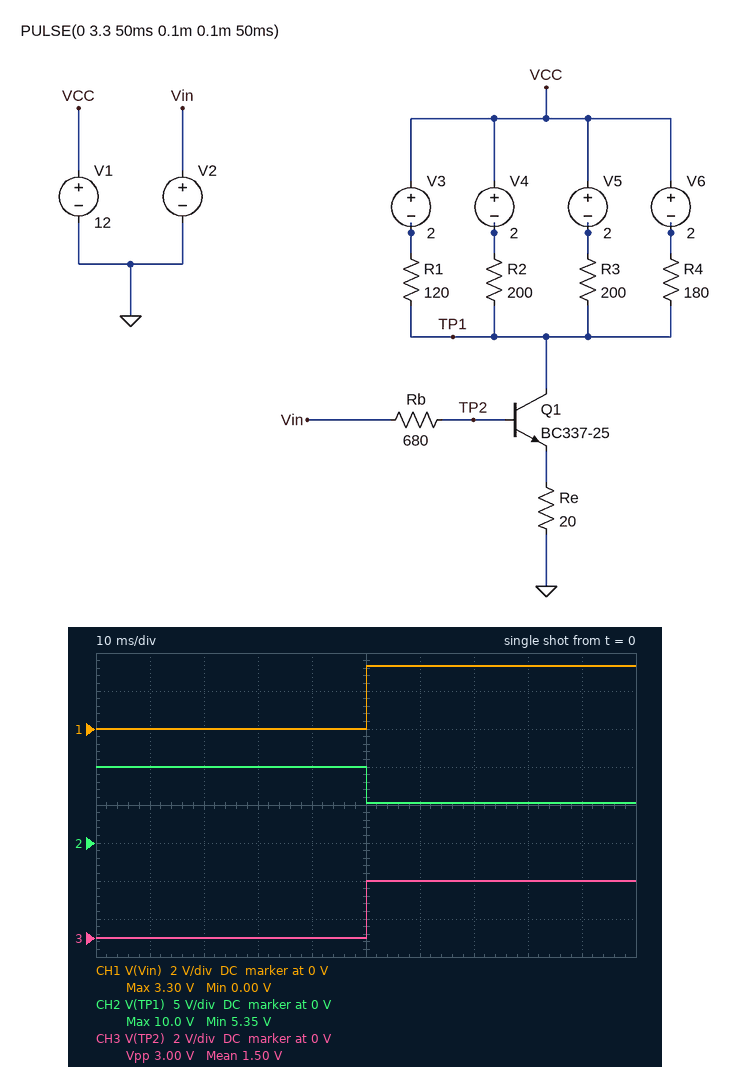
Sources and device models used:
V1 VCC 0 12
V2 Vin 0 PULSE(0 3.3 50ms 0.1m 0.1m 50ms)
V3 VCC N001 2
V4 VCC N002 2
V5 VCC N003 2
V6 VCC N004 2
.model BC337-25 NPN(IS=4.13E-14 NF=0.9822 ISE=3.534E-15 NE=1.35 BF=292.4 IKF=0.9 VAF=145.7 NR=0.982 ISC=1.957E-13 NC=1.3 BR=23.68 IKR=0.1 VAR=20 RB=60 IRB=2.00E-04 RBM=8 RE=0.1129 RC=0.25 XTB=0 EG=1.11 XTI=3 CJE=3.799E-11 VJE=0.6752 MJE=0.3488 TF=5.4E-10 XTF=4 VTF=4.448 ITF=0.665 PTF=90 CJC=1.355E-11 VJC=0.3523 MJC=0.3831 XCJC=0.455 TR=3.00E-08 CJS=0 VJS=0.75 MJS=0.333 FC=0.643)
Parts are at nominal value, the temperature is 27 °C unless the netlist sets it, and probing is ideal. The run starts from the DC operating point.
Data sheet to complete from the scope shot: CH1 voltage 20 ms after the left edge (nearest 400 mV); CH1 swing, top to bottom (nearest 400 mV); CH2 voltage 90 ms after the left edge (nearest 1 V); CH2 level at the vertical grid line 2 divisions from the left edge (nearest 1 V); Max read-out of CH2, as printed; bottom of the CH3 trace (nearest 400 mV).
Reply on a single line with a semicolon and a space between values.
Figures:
0 V; 3.2 V; 5 V; 10 V; 10.0 V; 0 V
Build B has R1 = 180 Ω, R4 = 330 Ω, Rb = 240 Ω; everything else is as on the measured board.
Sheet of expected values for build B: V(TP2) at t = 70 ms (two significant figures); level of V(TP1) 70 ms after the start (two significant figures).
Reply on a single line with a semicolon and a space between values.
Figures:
3.2 V; 3.5 V
